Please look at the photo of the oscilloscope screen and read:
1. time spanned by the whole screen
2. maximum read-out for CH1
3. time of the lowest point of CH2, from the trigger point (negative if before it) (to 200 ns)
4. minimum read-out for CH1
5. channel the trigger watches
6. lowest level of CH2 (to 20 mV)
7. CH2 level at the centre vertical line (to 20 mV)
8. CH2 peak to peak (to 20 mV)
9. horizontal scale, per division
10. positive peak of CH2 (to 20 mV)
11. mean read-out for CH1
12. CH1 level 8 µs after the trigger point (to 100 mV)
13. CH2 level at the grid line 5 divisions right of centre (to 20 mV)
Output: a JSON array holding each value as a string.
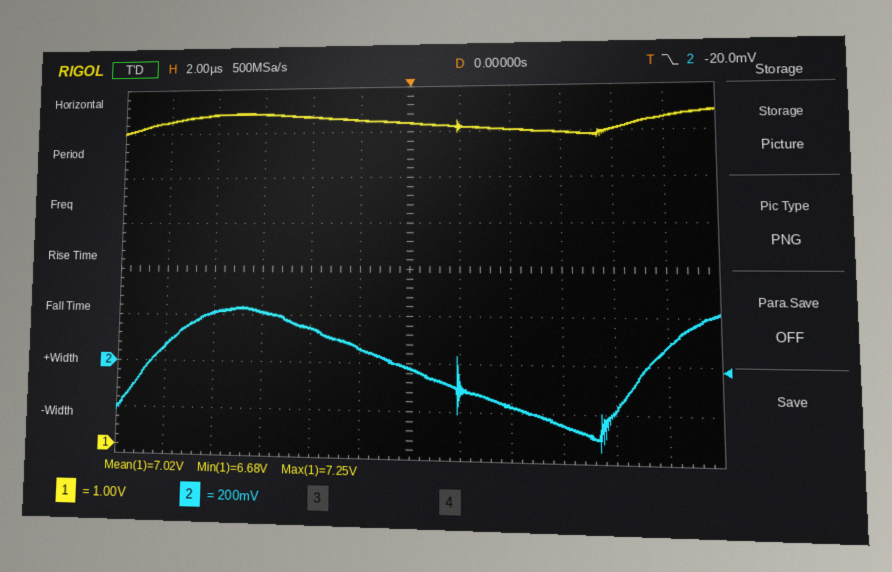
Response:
["24 µs", "7.25 V", "+7.4 µs", "6.68 V", "CH2", "-340 mV", "-20 mV", "580 mV", "2 µs", "240 mV", "7.02 V", "6.8 V", "80 mV"]
